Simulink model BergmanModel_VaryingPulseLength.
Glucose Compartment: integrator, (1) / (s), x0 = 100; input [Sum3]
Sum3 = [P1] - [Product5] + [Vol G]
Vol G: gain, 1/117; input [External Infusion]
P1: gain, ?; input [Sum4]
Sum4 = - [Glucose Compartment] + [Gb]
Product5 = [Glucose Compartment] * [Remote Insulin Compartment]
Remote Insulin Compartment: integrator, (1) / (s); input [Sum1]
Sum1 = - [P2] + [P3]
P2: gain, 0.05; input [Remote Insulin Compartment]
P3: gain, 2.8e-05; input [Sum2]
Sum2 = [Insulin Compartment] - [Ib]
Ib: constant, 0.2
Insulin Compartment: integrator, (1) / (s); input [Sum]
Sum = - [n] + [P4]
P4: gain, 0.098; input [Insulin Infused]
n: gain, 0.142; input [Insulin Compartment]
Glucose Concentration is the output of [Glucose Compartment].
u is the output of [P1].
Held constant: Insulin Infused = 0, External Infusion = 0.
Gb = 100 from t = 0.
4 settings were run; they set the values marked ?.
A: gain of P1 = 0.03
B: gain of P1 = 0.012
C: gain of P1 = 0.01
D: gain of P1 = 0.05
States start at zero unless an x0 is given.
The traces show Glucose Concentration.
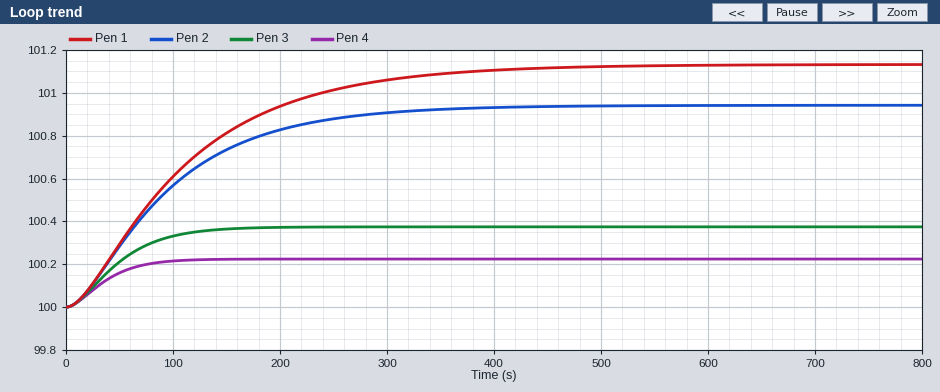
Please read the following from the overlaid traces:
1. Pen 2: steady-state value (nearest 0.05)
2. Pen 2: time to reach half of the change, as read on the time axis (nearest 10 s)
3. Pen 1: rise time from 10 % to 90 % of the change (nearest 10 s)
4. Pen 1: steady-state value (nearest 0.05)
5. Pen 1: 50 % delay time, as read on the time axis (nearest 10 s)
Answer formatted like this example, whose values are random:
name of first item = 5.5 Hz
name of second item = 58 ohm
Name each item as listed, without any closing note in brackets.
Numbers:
Pen 2: steady-state value = 100.95
Pen 2: time to reach half of the change, as read on the time axis = 80 s
Pen 1: rise time from 10 % to 90 % of the change = 230 s
Pen 1: steady-state value = 101.15
Pen 1: 50 % delay time, as read on the time axis = 90 s
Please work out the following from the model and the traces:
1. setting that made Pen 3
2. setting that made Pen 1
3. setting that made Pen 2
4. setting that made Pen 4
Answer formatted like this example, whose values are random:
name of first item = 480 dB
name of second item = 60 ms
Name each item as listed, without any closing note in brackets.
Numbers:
setting that made Pen 3 = A
setting that made Pen 1 = C
setting that made Pen 2 = B
setting that made Pen 4 = D
